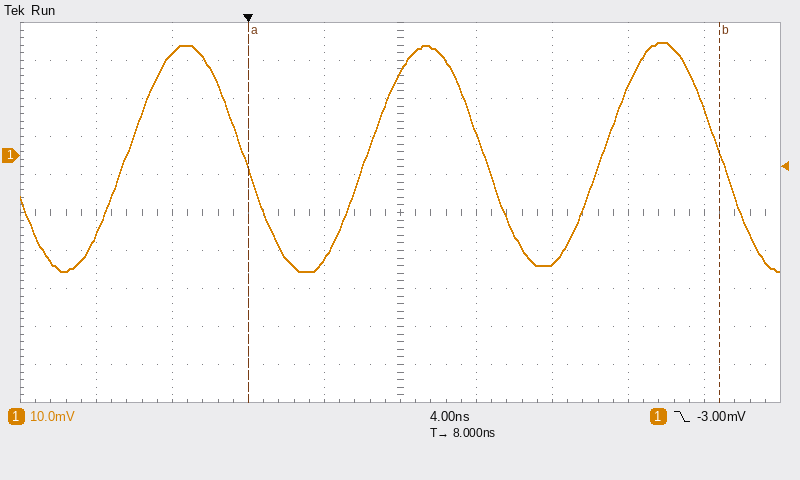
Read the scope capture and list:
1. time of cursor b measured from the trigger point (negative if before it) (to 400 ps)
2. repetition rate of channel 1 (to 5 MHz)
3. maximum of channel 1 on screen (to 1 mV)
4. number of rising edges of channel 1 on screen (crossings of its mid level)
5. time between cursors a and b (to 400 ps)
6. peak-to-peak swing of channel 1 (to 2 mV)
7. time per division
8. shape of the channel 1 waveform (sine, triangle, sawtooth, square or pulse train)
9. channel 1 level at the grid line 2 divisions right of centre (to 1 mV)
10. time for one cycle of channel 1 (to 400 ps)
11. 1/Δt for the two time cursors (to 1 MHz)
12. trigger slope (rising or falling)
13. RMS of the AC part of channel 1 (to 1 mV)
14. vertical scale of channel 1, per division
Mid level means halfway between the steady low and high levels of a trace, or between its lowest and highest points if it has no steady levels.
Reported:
+24.8 ns
80 MHz
30 mV
3
24.8 ns
60 mV
4 ns
sine
-28 mV
12.4 ns
40 MHz
falling
21 mV
10 mV
